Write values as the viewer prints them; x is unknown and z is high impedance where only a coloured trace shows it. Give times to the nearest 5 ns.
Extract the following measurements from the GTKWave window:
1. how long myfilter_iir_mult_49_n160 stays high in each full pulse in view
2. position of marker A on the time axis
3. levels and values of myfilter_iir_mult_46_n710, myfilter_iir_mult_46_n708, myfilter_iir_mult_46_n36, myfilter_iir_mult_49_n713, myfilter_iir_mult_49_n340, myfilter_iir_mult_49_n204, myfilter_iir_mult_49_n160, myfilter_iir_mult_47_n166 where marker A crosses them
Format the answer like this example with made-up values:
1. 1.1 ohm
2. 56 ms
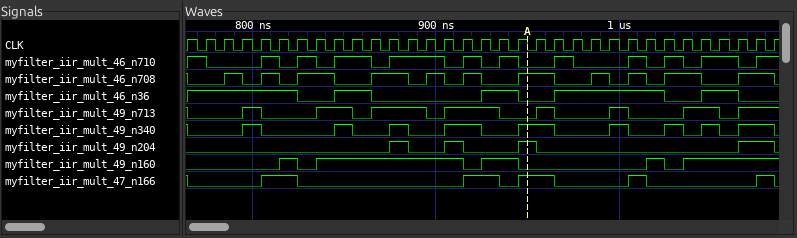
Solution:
1. 10 ns, 80 ns, 20 ns, 10 ns
2. 950 ns
3. myfilter_iir_mult_46_n710=0, myfilter_iir_mult_46_n708=1, myfilter_iir_mult_46_n36=0, myfilter_iir_mult_49_n713=0, myfilter_iir_mult_49_n340=1, myfilter_iir_mult_49_n204=1, myfilter_iir_mult_49_n160=0, myfilter_iir_mult_47_n166=1
